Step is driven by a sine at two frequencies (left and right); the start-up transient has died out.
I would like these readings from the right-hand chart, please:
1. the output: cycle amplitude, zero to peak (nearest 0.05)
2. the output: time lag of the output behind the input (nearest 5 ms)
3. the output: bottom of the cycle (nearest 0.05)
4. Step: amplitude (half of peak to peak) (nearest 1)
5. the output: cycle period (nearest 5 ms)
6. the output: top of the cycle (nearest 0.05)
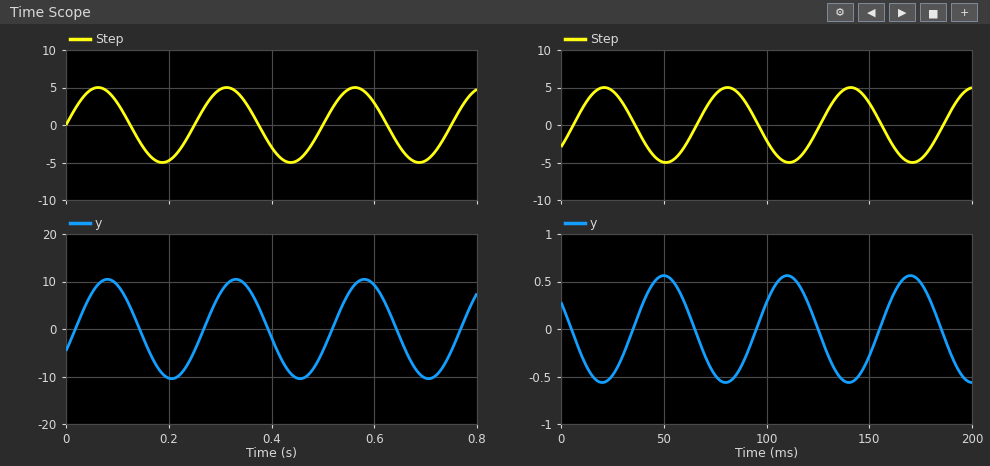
0.55
30 ms
-0.55
5
60 ms
0.55
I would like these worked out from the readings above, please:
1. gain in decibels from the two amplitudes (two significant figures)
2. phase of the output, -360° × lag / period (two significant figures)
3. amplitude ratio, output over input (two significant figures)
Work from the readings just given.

-19 dB
-180°
0.11
